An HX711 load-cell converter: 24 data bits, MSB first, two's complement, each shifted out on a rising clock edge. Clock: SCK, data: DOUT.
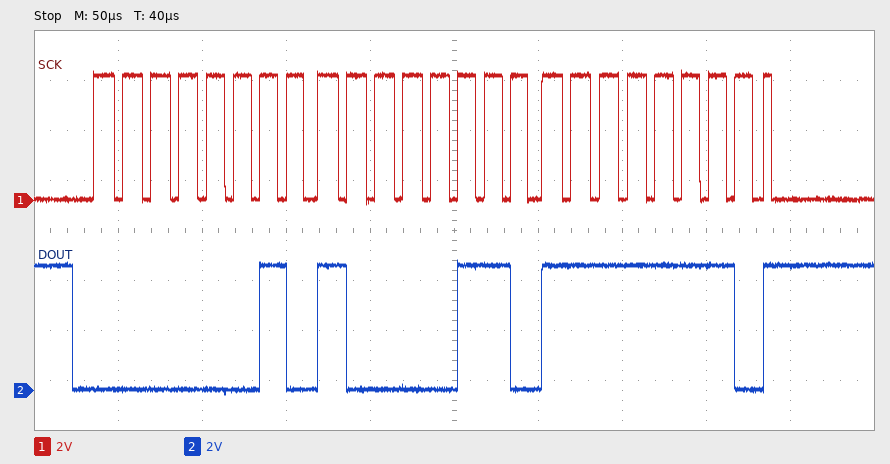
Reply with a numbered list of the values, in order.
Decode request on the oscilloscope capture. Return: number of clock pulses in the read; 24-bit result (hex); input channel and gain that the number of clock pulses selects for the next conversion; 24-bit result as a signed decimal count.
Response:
1. 25
2. 0x0286FE
3. channel A, gain 128
4. 165630
